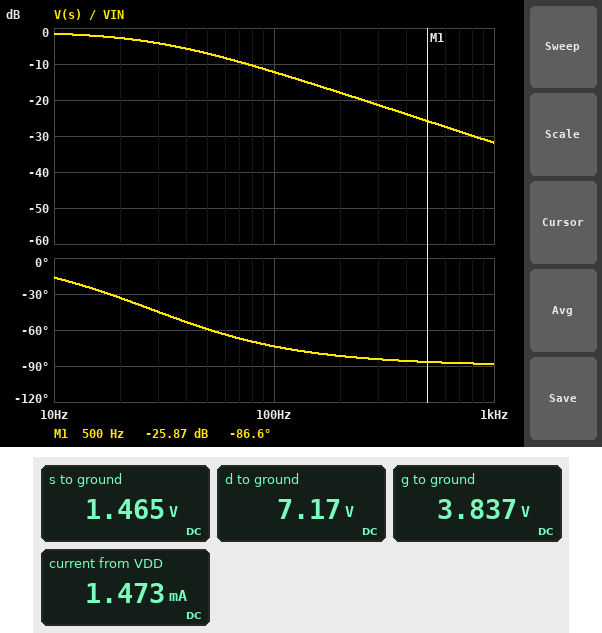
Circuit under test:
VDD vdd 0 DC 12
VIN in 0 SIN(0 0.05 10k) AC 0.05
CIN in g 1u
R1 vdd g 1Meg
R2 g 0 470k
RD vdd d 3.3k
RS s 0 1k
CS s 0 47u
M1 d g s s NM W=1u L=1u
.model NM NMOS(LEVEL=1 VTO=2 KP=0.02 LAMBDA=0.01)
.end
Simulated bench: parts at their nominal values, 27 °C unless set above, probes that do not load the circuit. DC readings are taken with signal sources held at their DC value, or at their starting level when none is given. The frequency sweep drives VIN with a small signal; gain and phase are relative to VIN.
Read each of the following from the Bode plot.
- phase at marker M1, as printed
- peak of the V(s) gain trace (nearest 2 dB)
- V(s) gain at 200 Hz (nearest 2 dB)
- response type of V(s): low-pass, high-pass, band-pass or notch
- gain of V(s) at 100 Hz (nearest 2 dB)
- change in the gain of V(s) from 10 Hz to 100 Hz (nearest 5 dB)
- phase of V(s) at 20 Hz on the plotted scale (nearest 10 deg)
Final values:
-86.6 deg
-2 dB
-18 dB
low-pass
-12 dB
-10 dB
-30 deg
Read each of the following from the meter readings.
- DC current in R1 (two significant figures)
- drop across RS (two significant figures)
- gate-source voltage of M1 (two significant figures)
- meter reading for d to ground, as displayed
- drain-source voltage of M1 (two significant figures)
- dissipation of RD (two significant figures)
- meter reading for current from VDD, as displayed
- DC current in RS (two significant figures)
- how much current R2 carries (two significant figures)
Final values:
8.2 µA
1.5 V
2.4 V
7.17 V
5.7 V
7.1 mW
1.473 mA
1.5 mA
8.2 µA
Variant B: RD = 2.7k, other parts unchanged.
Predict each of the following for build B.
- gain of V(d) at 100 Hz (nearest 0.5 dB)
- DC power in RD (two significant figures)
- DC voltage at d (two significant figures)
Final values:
26.0 dB
5.8 mW
8.0 V
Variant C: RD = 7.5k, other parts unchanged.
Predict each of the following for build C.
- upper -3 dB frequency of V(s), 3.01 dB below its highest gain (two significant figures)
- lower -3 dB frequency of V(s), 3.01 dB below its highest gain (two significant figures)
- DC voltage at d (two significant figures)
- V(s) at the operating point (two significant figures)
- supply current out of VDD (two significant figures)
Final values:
5.1 Hz
410 mHz
1.6 V
1.4 V
1.4 mA
